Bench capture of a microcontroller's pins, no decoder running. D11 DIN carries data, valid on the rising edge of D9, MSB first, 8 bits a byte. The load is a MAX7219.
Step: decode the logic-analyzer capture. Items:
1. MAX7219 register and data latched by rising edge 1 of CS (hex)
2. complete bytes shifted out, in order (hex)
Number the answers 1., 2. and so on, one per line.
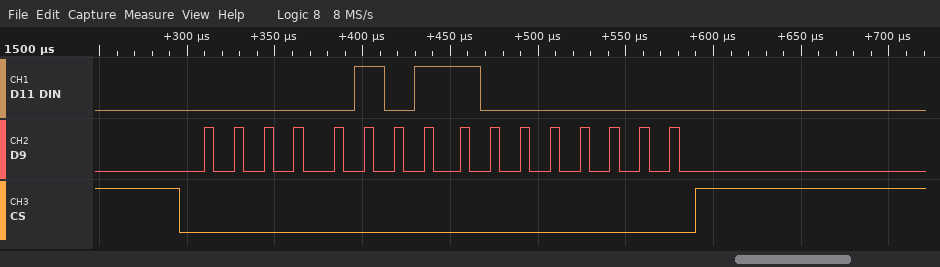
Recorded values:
1. register 0x5, data 0x80
2. 0x05 0x80
